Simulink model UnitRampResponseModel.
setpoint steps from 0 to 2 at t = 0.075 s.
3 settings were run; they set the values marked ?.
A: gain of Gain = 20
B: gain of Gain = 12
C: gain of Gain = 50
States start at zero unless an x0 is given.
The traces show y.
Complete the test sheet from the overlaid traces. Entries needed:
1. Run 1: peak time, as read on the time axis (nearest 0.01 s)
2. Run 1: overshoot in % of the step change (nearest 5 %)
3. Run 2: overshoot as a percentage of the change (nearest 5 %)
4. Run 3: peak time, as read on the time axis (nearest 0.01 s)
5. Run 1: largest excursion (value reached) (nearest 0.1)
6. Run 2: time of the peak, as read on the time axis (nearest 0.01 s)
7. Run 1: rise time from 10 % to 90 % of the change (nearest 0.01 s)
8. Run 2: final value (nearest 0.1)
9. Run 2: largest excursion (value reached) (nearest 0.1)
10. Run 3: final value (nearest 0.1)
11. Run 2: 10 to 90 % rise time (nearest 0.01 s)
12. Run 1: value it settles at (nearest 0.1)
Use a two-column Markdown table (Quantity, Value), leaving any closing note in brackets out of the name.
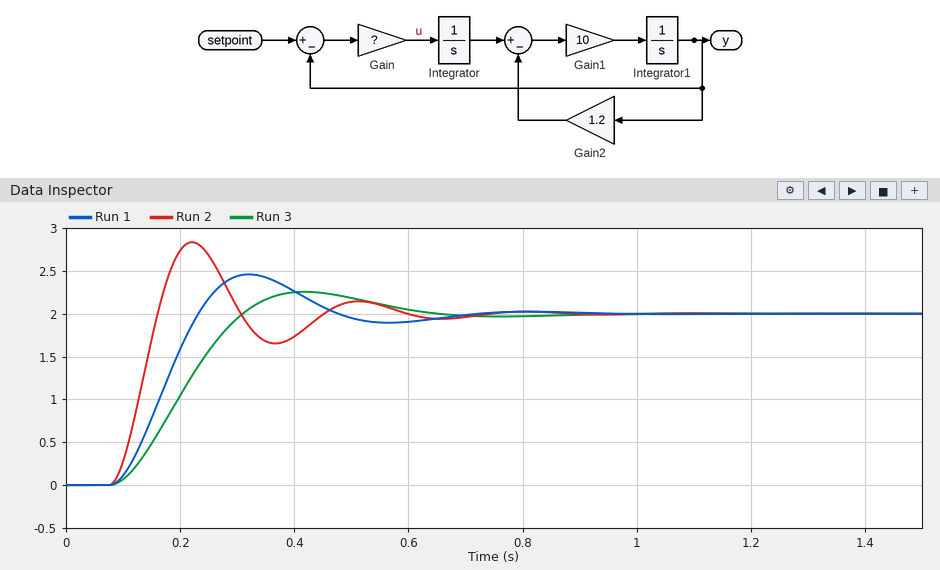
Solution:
| Quantity | Value |
|---|---|
| Run 1: peak time, as read on the time axis | 0.32 s |
| Run 1: overshoot in % of the step change | 25 % |
| Run 2: overshoot as a percentage of the change | 40 % |
| Run 3: peak time, as read on the time axis | 0.42 s |
| Run 1: largest excursion (value reached) | 2.5 |
| Run 2: time of the peak, as read on the time axis | 0.22 s |
| Run 1: rise time from 10 % to 90 % of the change | 0.11 s |
| Run 2: final value | 2.0 |
| Run 2: largest excursion (value reached) | 2.8 |
| Run 3: final value | 2.0 |
| Run 2: 10 to 90 % rise time | 0.06 s |
| Run 1: value it settles at | 2.0 |
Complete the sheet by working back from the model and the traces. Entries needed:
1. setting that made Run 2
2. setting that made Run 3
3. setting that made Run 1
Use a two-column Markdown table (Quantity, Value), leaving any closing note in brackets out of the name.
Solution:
| Quantity | Value |
|---|---|
| setting that made Run 2 | C |
| setting that made Run 3 | B |
| setting that made Run 1 | A |
